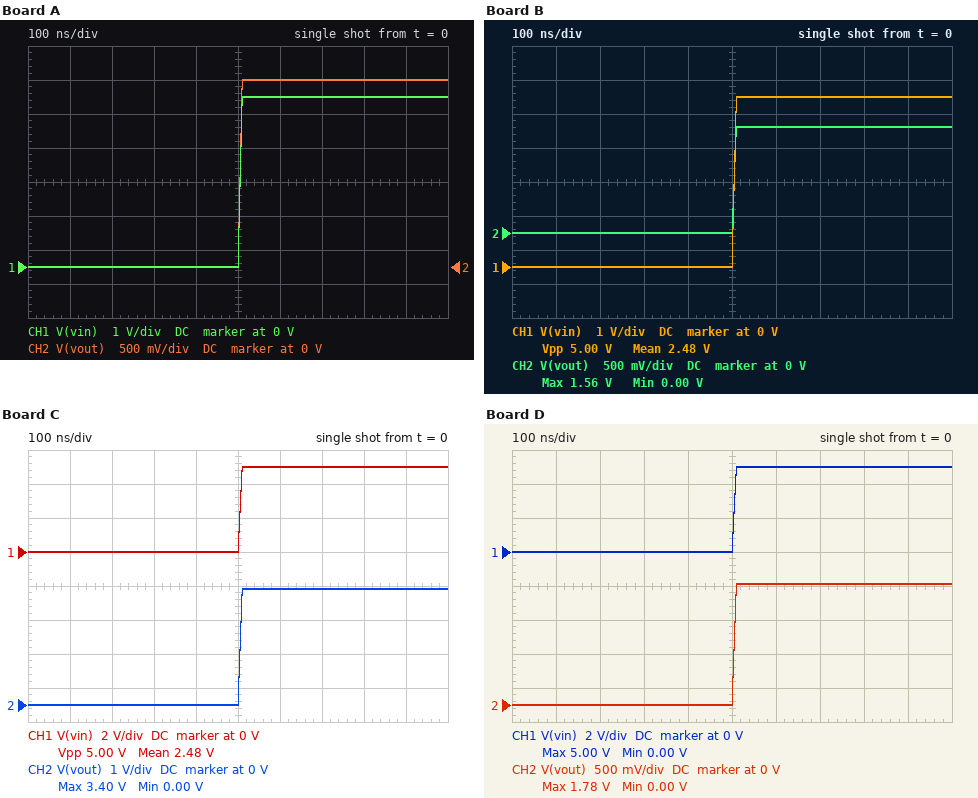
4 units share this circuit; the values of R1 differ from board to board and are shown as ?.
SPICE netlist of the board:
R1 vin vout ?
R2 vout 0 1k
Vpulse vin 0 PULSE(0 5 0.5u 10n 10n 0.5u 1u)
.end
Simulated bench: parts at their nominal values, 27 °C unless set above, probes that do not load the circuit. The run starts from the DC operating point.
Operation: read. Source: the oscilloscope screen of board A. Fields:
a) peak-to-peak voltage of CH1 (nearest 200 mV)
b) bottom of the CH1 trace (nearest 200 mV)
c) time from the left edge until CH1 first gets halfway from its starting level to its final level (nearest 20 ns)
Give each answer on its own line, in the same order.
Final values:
5.0 V
0 V
500 ns
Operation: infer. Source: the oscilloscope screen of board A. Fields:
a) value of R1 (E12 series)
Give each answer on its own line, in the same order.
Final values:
820 Ω
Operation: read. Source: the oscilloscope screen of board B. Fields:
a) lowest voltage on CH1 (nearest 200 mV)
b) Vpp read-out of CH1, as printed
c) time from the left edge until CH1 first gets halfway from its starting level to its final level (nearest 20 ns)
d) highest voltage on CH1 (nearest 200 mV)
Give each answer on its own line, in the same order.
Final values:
0 V
5.00 V
500 ns
5.0 V
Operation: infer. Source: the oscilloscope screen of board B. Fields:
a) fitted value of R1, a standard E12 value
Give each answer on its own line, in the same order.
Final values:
2.2 kΩ
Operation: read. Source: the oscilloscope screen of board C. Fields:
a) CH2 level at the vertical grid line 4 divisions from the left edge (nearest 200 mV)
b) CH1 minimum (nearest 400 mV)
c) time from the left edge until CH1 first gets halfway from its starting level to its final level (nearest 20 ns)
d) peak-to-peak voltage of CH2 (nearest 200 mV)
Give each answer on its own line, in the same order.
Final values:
0 V
0 V
500 ns
3.4 V
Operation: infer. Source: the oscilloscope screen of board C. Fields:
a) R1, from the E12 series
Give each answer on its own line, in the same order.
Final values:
470 Ω
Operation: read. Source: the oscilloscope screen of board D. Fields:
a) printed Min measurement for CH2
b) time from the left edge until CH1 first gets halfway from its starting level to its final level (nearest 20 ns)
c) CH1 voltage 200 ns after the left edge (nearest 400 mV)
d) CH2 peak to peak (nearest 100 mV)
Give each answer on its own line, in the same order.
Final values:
0.00 V
500 ns
0 V
1.8 V
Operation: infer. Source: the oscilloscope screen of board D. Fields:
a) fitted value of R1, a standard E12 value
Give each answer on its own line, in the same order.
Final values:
1.8 kΩ
